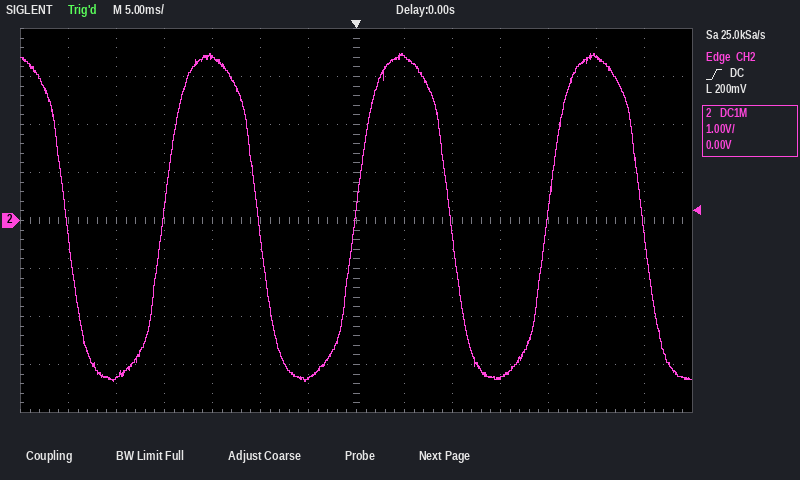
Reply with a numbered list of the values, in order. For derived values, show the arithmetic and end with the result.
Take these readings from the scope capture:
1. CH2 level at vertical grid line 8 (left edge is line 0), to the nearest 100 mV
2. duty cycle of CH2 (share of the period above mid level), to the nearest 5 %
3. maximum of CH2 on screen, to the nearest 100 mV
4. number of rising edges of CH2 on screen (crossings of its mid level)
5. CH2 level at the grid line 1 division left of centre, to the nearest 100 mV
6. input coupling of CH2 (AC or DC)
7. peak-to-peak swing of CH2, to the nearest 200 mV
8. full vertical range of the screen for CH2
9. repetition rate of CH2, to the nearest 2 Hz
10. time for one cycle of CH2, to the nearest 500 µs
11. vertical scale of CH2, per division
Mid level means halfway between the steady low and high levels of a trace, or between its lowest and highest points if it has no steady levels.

1. 3.4 V
2. 50 %
3. 3.5 V
4. 3
5. -3.3 V
6. DC
7. 6.8 V
8. 8 V
9. 1 / 20.0 ms ≈ 50 Hz
10. 20.0 ms
11. 1 V
